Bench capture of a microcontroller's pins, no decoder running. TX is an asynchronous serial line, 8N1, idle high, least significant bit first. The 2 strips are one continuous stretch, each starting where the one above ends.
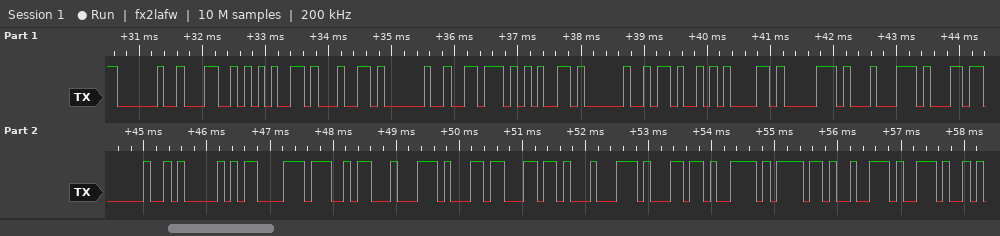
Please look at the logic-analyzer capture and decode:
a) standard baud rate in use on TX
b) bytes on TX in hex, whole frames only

9600 baud
20 4C 65 64 20 76 65 20 4B 61 70 C4 B1 20 41 C3 A7 C4 B1 6C C4 B1 79 6F 72 2E
